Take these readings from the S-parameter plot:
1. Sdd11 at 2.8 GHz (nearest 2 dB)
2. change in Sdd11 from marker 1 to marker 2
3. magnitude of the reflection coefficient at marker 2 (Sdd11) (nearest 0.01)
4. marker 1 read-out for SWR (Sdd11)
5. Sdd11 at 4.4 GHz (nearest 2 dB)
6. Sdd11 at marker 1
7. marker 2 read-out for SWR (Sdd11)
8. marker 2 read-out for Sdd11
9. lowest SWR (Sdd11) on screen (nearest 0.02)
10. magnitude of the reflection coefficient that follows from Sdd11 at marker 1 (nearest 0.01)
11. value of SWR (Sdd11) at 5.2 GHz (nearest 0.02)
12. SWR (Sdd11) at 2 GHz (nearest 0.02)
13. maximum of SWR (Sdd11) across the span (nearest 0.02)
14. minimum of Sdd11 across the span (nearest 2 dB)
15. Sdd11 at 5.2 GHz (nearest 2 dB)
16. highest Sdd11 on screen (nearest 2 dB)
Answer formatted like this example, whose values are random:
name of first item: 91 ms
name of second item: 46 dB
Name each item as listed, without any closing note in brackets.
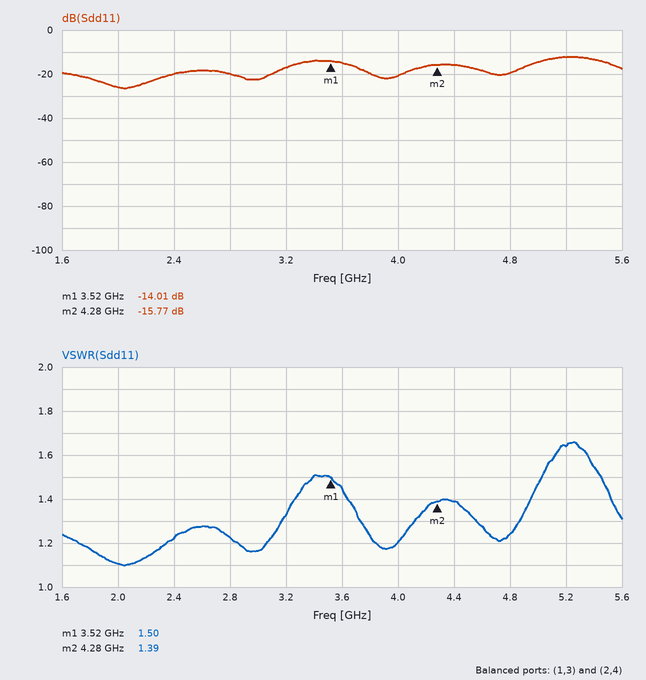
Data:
Sdd11 at 2.8 GHz: -20 dB
change in Sdd11 from marker 1 to marker 2: -1.76 dB
magnitude of the reflection coefficient at marker 2 (Sdd11): 0.16
marker 1 read-out for SWR: 1.50
Sdd11 at 4.4 GHz: -16 dB
Sdd11 at marker 1: -14.01 dB
marker 2 read-out for SWR: 1.39
marker 2 read-out for Sdd11: -15.77 dB
lowest SWR (Sdd11) on screen: 1.10
magnitude of the reflection coefficient that follows from Sdd11 at marker 1: 0.20
value of SWR (Sdd11) at 5.2 GHz: 1.64
SWR (Sdd11) at 2 GHz: 1.10
maximum of SWR (Sdd11) across the span: 1.66
minimum of Sdd11 across the span: -26 dB
Sdd11 at 5.2 GHz: -12 dB
highest Sdd11 on screen: -12 dB
